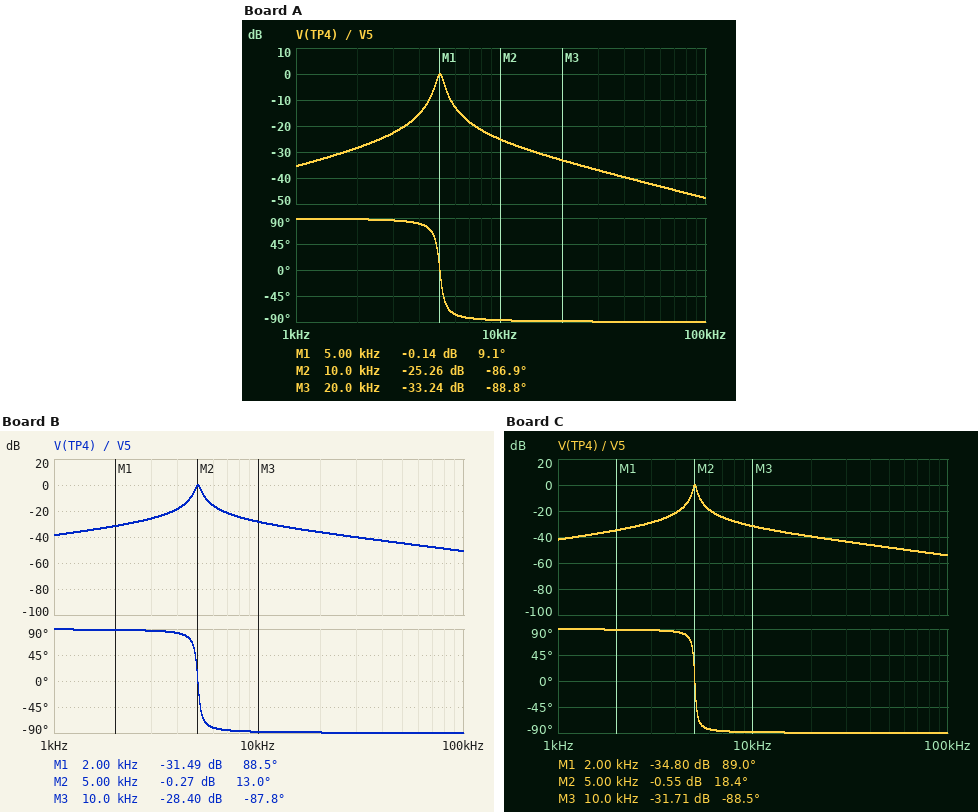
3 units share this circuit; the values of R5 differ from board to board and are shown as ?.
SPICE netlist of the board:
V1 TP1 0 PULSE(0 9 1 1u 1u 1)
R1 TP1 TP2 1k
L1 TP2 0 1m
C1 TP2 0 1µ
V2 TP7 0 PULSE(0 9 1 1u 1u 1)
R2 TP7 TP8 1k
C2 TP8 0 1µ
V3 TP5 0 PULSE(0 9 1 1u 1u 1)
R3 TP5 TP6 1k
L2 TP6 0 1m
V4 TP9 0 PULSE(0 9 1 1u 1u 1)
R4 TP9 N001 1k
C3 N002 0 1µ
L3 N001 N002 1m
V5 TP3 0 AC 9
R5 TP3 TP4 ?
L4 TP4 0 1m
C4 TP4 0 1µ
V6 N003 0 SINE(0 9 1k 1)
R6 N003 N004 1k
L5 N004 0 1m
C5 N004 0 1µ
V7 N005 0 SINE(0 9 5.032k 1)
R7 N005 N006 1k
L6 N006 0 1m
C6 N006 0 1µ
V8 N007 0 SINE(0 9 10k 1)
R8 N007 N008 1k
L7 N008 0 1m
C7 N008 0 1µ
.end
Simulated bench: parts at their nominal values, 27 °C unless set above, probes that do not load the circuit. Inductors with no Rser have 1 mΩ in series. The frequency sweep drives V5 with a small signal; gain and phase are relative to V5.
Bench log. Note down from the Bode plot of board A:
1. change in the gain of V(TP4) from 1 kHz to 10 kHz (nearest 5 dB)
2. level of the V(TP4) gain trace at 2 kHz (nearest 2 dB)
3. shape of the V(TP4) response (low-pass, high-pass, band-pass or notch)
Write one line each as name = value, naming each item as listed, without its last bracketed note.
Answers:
change in the gain of V(TP4) from 1 kHz to 10 kHz = 10 dB
level of the V(TP4) gain trace at 2 kHz = -28 dB
shape of the V(TP4) response = band-pass
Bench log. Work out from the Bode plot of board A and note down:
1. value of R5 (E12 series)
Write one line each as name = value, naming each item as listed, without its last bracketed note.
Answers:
value of R5 = 390 Ω
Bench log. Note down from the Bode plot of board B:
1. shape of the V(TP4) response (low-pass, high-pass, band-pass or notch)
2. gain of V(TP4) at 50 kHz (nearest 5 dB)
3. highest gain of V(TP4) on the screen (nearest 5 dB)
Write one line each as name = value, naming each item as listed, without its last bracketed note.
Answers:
shape of the V(TP4) response = band-pass
gain of V(TP4) at 50 kHz = -45 dB
highest gain of V(TP4) on the screen = 0 dB
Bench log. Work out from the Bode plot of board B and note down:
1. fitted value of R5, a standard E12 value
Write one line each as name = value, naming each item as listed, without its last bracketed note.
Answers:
fitted value of R5, a standard E12 value = 560 Ω
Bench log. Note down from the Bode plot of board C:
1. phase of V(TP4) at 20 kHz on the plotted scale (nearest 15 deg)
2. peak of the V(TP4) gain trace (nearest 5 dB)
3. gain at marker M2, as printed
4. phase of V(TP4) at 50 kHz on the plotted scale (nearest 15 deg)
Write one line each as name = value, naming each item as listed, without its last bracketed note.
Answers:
phase of V(TP4) at 20 kHz on the plotted scale = -90 deg
peak of the V(TP4) gain trace = 0 dB
gain at marker M2, as printed = -0.55 dB
phase of V(TP4) at 50 kHz on the plotted scale = -90 deg
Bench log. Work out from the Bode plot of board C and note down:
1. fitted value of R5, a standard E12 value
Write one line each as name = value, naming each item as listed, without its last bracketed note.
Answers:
fitted value of R5, a standard E12 value = 820 Ω
